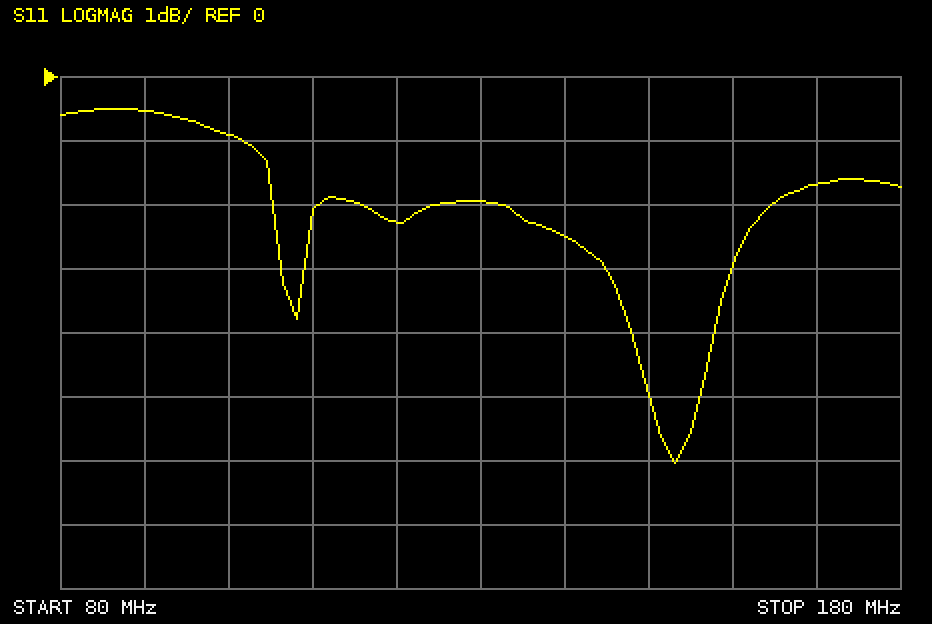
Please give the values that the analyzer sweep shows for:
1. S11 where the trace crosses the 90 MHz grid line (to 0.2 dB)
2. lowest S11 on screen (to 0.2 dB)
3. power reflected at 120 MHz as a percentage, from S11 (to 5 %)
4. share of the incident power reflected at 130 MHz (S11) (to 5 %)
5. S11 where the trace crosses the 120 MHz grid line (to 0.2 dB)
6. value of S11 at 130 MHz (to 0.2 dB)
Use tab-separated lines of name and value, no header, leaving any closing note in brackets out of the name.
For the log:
S11 where the trace crosses the 90 MHz grid line	-0.6 dB
lowest S11 on screen	-6.0 dB
power reflected at 120 MHz as a percentage, from S11	60 %
share of the incident power reflected at 130 MHz (S11)	65 %
S11 where the trace crosses the 120 MHz grid line	-2.2 dB
value of S11 at 130 MHz	-2.0 dB
